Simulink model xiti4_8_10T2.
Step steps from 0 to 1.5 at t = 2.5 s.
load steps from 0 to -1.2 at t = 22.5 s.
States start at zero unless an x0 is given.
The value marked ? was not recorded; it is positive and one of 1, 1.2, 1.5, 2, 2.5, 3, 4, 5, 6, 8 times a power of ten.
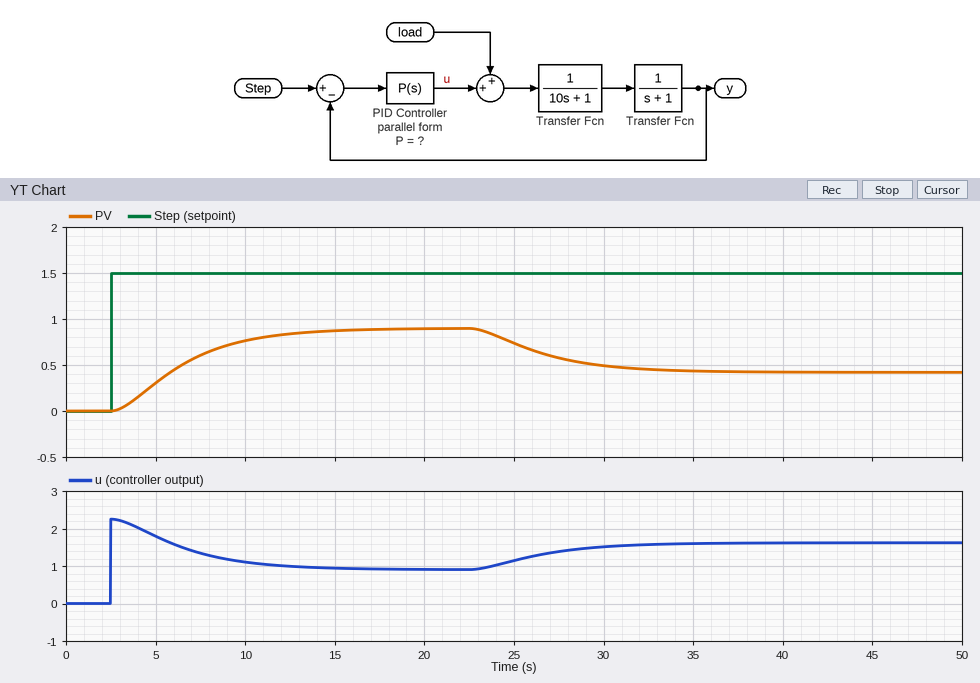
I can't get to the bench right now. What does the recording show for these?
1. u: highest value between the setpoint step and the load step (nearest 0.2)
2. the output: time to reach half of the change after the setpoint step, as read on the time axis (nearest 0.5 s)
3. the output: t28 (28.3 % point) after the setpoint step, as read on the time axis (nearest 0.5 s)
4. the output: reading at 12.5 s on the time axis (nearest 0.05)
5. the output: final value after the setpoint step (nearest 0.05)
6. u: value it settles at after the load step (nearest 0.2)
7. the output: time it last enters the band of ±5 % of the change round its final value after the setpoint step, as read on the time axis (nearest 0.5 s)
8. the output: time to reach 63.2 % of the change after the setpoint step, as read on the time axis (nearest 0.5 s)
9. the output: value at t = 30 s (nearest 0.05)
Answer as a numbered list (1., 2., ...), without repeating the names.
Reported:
1. 2.2
2. 6.0 s
3. 4.5 s
4. 0.85
5. 0.90
6. 1.6
7. 13.5 s
8. 7.0 s
9. 0.50
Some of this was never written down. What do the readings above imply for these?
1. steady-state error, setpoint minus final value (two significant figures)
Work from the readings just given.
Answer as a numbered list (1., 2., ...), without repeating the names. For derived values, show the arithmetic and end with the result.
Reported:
1. 1.5 - 0.9 = 0.60
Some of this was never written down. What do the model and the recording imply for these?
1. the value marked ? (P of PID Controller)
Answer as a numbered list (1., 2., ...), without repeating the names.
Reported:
1. 1.5
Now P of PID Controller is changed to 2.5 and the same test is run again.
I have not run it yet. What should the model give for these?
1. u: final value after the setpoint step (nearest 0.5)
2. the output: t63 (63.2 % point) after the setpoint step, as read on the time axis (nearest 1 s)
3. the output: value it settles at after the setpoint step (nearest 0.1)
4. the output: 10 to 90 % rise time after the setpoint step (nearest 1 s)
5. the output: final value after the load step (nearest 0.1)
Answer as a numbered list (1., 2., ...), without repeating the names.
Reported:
1. 1.0
2. 6 s
3. 1.1
4. 5 s
5. 0.7
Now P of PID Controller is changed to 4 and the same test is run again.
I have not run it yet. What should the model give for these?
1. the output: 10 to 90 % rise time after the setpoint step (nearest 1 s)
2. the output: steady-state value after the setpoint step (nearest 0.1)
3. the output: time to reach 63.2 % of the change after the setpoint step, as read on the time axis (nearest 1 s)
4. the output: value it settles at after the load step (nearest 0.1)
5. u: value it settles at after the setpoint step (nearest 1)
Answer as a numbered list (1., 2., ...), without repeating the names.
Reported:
1. 3 s
2. 1.2
3. 5 s
4. 1.0
5. 1
